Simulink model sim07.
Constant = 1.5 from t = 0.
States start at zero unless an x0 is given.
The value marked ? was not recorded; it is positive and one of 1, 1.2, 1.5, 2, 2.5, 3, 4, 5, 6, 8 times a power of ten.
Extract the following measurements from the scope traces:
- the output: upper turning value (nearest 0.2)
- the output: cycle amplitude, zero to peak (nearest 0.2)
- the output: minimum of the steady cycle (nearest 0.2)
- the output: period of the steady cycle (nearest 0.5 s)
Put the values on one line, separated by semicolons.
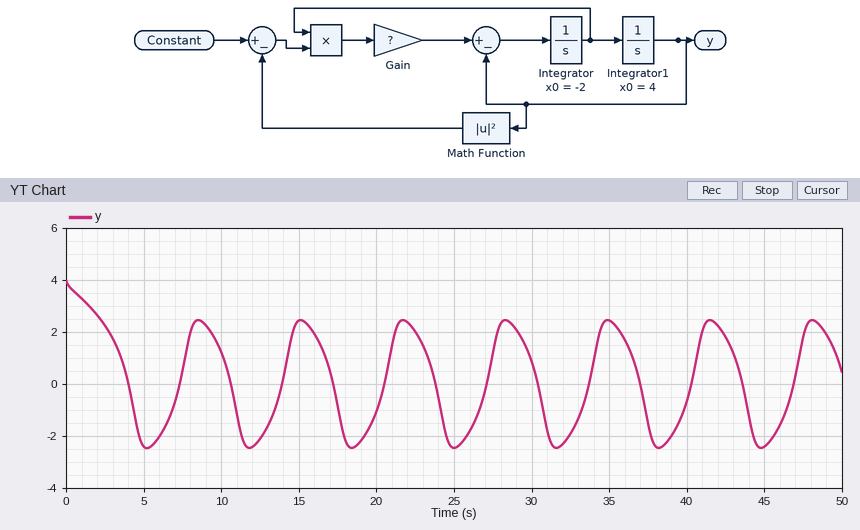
2.4; 2.4; -2.4; 6.5 s
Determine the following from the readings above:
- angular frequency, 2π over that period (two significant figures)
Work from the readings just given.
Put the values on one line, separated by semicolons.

0.97 rad/s
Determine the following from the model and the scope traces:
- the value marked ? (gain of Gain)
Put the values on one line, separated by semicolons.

0.6
